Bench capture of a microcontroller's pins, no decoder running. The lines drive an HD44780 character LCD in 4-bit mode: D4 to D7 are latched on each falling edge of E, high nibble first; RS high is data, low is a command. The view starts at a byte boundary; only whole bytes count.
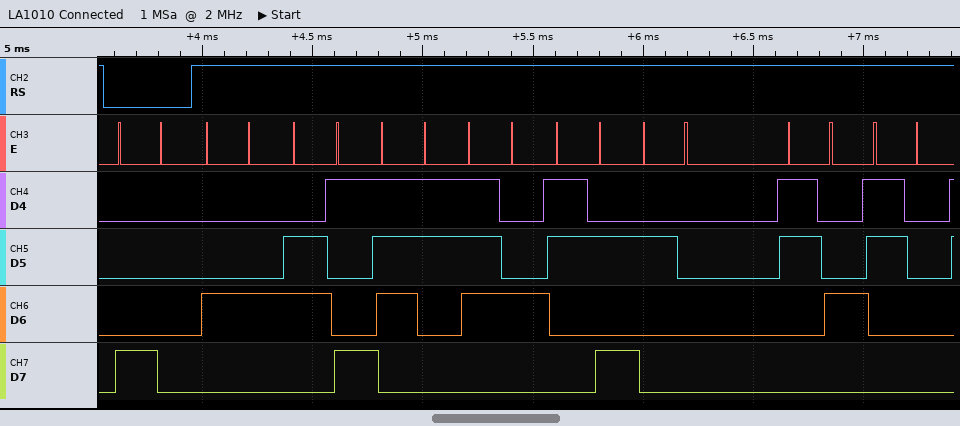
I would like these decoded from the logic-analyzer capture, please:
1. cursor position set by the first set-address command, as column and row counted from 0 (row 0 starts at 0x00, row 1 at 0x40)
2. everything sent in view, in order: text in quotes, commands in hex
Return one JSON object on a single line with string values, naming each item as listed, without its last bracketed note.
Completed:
{"cursor position set by the first set-address command, as column and row counted from 0": "column 0, row 0", "everything sent in view, in order: text in quotes, commands in hex": "0x80 \"Dist: 40\""}
